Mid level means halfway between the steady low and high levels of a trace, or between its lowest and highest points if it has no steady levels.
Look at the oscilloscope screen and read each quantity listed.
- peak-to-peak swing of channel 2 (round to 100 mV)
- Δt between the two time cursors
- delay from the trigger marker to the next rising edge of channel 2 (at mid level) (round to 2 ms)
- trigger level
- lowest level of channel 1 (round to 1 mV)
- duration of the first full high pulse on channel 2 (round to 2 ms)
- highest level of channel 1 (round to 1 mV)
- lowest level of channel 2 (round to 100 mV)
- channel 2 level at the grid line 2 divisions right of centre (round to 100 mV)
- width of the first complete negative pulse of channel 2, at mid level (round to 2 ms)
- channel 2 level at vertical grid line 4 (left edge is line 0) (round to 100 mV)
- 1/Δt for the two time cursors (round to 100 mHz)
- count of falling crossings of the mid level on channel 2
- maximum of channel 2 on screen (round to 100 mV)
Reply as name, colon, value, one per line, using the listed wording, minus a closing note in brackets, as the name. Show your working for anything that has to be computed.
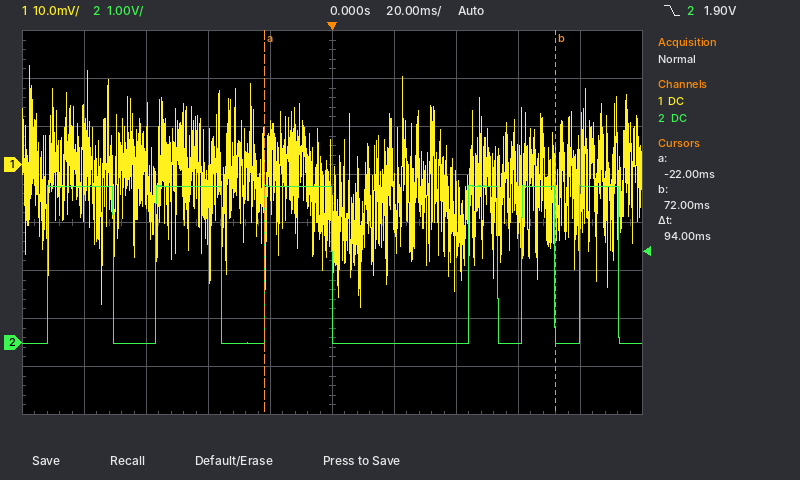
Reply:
peak-to-peak swing of channel 2: 3.3 V − (0.0 V) = 3.3 V
Δt between the two time cursors: 94 ms
delay from the trigger marker to the next rising edge of channel 2 (at mid level): 44 ms
trigger level: 1.90 V
lowest level of channel 1: -30 mV
duration of the first full high pulse on channel 2: 22 ms
highest level of channel 1: 21 mV
lowest level of channel 2: 0.0 V
channel 2 level at the grid line 2 divisions right of centre: 0.0 V
width of the first complete negative pulse of channel 2, at mid level: 14 ms
channel 2 level at vertical grid line 4 (left edge is line 0): 3.3 V
1/Δt for the two time cursors: 1 / 94 ms ≈ 10.6 Hz
count of falling crossings of the mid level on channel 2: 6
maximum of channel 2 on screen: 3.3 V
